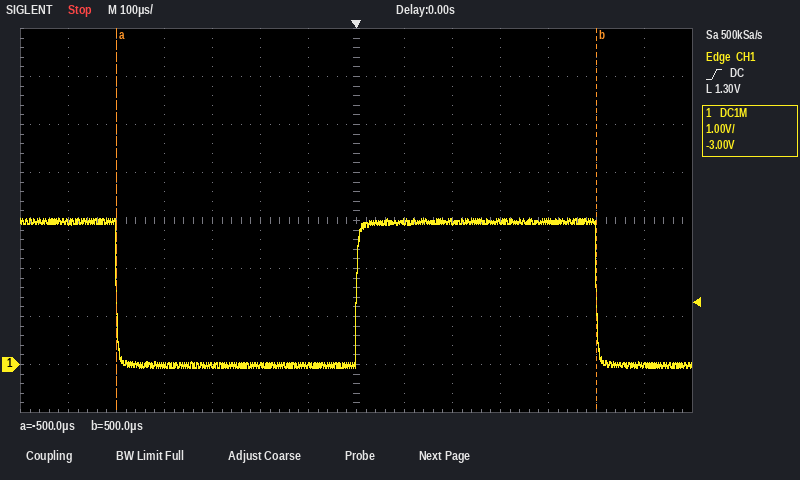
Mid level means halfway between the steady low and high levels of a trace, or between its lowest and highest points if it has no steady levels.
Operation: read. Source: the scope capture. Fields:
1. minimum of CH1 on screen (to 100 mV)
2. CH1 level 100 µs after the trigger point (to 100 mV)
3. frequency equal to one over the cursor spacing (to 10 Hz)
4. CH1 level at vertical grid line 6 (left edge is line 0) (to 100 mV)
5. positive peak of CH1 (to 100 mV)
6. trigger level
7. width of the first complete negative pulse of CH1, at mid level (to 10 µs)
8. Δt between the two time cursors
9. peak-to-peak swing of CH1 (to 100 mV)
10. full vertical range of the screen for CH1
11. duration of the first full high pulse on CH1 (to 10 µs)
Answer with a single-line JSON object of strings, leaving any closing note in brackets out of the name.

{"minimum of CH1 on screen": "-100 mV", "CH1 level 100 µs after the trigger point": "3.0 V", "frequency equal to one over the cursor spacing": "1.00 kHz", "CH1 level at vertical grid line 6 (left edge is line 0)": "0.0 V", "positive peak of CH1": "3.0 V", "trigger level": "1.30 V", "width of the first complete negative pulse of CH1, at mid level": "500 µs", "Δt between the two time cursors": "1.00 ms", "peak-to-peak swing of CH1": "3.1 V", "full vertical range of the screen for CH1": "8 V", "duration of the first full high pulse on CH1": "500 µs"}
